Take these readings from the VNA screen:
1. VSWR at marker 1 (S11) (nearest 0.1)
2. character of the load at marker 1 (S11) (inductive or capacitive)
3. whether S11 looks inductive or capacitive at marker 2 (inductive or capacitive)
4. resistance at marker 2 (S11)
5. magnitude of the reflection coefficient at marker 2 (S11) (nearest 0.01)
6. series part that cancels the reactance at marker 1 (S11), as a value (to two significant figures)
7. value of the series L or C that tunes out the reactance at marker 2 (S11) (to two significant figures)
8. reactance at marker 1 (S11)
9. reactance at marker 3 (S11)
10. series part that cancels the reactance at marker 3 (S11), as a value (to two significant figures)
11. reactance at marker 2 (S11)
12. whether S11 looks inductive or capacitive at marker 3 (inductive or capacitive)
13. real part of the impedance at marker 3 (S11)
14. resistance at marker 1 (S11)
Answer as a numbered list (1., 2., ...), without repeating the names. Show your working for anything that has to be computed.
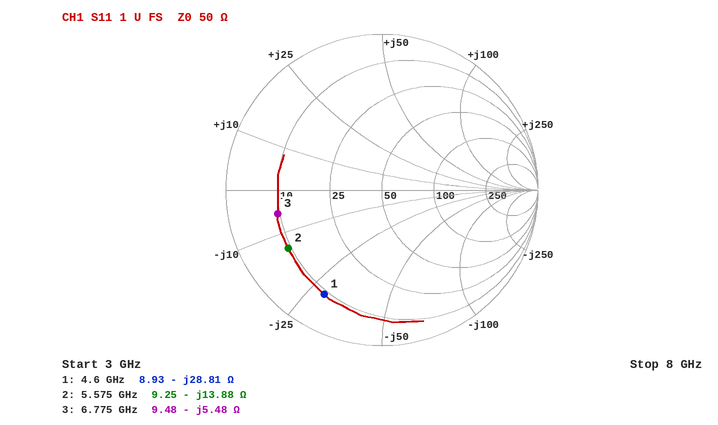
1. 7.5
2. capacitive
3. capacitive
4. 9.25 Ω
5. 0.71
6. L = 28.81 Ω/(2π × 4.6 GHz) ≈ 1.00 nH
7. L = 13.88 Ω/(2π × 5.575 GHz) ≈ 396 pH, so 400 pH to two significant figures
8. -28.81 Ω
9. -5.48 Ω
10. L = 5.48 Ω/(2π × 6.775 GHz) ≈ 129 pH, so 130 pH to two significant figures
11. -13.88 Ω
12. capacitive
13. 9.48 Ω
14. 8.93 Ω
